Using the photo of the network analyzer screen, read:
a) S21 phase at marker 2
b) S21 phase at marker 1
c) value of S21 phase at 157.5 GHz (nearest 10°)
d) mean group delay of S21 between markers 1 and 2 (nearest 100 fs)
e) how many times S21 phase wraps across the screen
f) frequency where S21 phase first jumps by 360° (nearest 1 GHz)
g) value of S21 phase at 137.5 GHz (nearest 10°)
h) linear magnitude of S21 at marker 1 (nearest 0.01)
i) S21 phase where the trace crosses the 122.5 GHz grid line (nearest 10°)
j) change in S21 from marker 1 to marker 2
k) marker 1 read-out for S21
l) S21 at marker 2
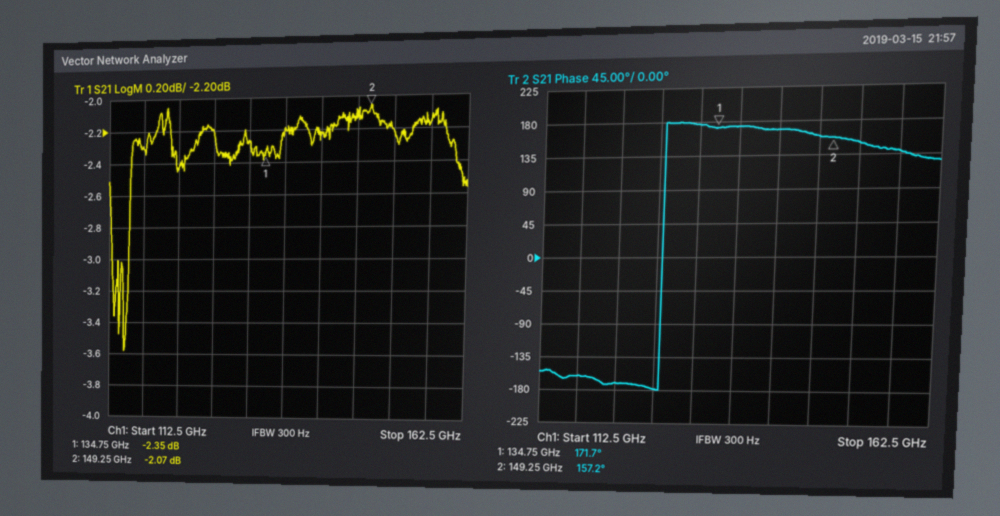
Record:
157.2°
171.7°
140°
2.8 ps
1
128 GHz
170°
0.76
-170°
0.28 dB
-2.35 dB
-2.07 dB
